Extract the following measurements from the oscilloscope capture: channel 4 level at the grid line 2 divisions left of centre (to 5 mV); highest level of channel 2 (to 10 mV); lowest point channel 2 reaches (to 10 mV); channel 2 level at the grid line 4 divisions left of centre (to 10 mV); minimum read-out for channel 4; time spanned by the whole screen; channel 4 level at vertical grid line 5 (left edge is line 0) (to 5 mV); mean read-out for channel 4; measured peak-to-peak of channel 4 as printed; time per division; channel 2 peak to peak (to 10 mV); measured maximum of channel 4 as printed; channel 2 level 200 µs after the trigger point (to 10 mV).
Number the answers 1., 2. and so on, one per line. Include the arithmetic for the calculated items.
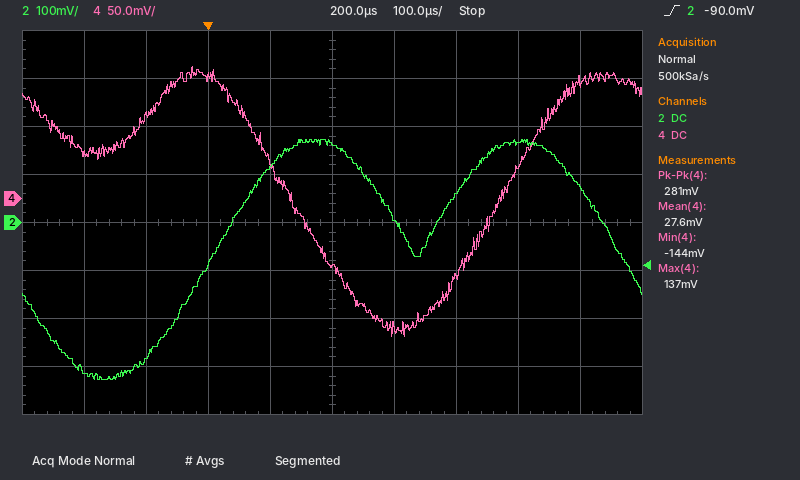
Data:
1. 125 mV
2. 170 mV
3. -330 mV
4. -310 mV
5. -144 mV
6. 1 ms
7. -70 mV
8. 27.6 mV
9. 281 mV
10. 100 µs
11. 170 mV − (-330 mV) = 500 mV
12. 137 mV
13. 170 mV
